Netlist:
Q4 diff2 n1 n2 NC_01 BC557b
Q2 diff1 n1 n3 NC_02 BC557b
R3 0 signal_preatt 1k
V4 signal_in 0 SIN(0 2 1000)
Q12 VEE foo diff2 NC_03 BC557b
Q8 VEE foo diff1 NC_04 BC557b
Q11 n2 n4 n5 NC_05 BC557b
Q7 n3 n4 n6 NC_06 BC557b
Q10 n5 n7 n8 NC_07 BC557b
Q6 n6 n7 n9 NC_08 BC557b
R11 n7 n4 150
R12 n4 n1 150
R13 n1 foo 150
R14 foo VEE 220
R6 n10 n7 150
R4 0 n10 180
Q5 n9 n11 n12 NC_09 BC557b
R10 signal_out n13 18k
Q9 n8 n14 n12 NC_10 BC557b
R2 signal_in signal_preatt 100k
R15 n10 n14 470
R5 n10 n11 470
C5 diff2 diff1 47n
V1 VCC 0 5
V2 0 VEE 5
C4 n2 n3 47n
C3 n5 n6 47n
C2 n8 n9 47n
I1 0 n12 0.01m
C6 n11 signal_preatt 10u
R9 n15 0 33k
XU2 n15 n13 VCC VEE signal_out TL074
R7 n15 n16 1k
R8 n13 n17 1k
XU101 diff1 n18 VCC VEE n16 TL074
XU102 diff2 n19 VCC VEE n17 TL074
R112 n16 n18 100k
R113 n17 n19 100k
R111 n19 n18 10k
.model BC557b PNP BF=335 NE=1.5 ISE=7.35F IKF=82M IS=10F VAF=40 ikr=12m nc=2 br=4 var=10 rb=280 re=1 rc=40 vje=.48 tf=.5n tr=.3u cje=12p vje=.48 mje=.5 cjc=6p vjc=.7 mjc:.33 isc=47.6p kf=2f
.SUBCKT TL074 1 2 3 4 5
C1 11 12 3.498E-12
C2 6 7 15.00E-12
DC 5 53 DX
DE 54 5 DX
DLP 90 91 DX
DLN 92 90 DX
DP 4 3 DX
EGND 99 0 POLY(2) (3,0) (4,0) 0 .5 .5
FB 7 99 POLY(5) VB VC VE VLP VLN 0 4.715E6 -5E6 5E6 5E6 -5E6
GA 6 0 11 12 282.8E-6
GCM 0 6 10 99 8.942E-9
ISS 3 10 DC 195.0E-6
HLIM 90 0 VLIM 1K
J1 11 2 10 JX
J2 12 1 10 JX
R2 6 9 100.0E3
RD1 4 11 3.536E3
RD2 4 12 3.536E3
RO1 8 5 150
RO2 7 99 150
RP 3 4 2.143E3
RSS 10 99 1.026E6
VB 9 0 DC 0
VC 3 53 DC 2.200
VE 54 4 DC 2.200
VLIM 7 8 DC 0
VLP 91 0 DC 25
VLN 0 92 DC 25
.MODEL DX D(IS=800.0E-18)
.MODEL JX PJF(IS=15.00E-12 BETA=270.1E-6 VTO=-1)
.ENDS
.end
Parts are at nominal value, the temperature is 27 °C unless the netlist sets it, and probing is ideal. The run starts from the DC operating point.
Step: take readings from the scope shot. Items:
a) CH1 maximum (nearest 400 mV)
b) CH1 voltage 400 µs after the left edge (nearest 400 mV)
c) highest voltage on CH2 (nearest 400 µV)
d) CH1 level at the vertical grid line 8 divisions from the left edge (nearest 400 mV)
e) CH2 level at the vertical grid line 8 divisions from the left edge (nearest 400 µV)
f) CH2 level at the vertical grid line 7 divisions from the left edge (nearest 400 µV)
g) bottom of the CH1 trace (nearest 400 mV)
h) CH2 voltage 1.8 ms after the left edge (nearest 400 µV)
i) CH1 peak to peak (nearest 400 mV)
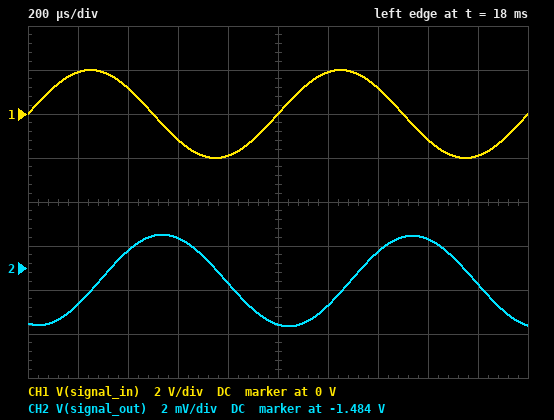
2.0 V
1.2 V
-1.4824 V
-1.2 V
-1.4828 V
-1.4832 V
-2.0 V
-1.4848 V
4.0 V
